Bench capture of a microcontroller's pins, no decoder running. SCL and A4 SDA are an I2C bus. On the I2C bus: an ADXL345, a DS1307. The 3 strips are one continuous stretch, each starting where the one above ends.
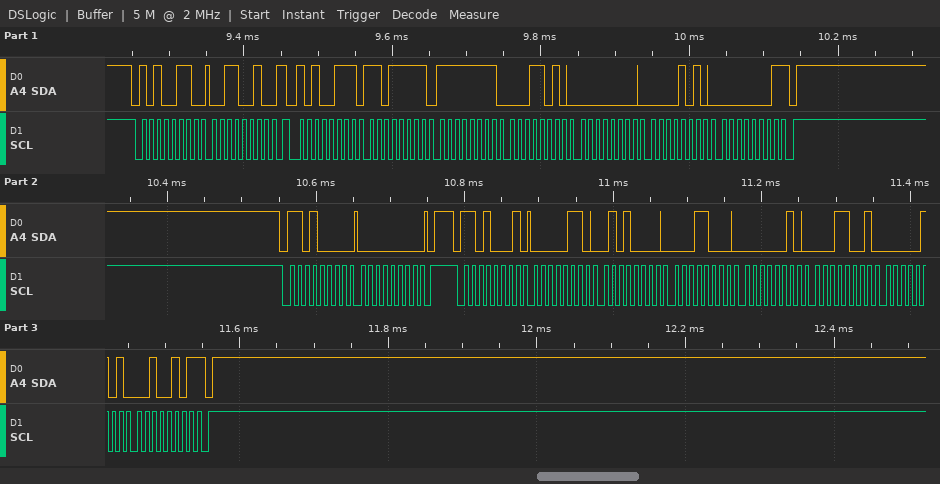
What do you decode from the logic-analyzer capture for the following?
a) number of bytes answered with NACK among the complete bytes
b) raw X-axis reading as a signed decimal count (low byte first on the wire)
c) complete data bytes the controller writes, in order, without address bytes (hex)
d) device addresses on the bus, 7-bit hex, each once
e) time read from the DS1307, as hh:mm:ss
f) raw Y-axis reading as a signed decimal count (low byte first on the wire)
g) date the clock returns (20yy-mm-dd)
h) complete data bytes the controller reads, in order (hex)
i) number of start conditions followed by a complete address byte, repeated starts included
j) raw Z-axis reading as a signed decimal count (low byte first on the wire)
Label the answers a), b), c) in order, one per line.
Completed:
a) 2
b) -33
c) 32 00
d) 0x53 0x68
e) 18:50:06
f) 26
g) 2025-05-19
h) DF FF 1A 00 0A 01 06 50 18 02 19 05 25
i) 4
j) 266
